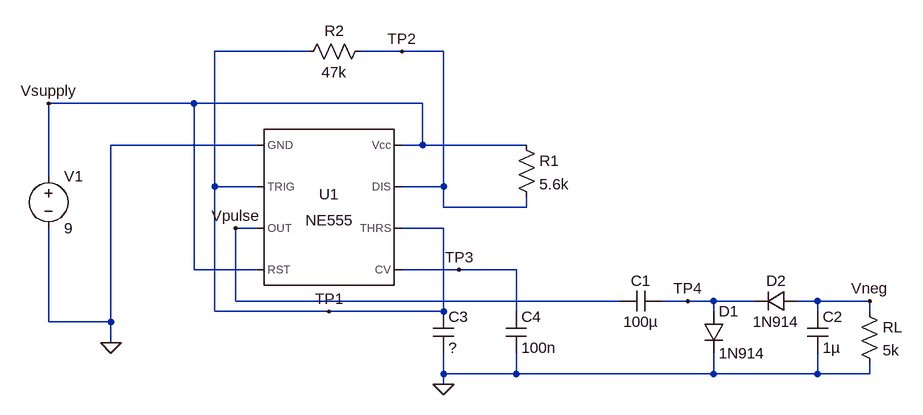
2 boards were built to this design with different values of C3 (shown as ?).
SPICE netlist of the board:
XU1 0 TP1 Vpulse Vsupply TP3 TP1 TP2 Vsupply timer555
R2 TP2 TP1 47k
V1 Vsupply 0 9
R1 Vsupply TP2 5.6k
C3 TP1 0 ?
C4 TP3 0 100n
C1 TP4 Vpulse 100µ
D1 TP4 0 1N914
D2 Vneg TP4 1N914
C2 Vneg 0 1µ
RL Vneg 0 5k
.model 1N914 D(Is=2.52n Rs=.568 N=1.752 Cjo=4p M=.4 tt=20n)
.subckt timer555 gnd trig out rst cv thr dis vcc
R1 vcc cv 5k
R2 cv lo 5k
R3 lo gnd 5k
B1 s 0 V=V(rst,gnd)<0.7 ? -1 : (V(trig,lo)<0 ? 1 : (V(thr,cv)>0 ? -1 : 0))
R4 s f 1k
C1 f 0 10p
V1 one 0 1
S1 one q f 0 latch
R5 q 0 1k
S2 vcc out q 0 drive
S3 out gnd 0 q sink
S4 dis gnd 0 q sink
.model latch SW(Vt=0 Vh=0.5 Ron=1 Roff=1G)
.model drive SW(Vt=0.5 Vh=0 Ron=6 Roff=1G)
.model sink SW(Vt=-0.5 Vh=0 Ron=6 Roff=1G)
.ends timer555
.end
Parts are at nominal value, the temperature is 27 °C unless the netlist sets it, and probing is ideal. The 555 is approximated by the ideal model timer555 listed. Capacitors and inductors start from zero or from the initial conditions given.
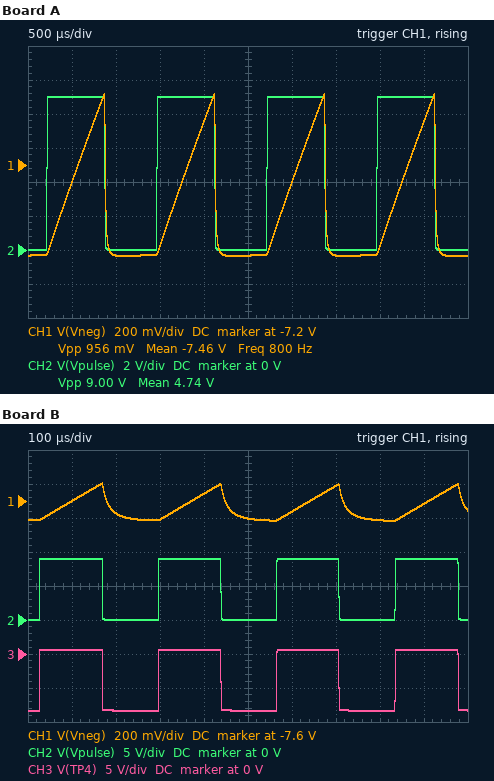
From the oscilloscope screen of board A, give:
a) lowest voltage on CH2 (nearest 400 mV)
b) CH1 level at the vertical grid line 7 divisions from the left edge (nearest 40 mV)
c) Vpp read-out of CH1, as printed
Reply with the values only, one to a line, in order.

0 V
-7.72 V
956 mV
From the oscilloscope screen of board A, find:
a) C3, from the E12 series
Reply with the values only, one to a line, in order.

18 nF
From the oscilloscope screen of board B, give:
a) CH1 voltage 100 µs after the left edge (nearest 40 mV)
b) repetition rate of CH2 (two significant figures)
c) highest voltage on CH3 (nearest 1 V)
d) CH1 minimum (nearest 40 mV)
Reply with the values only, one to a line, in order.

-7.60 V
3.7 kHz
1 V
-7.72 V
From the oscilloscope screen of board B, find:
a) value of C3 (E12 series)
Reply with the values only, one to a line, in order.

3.9 nF
